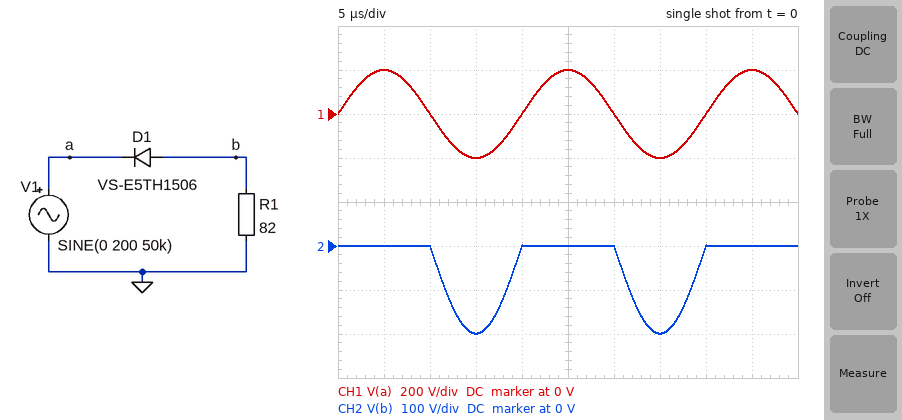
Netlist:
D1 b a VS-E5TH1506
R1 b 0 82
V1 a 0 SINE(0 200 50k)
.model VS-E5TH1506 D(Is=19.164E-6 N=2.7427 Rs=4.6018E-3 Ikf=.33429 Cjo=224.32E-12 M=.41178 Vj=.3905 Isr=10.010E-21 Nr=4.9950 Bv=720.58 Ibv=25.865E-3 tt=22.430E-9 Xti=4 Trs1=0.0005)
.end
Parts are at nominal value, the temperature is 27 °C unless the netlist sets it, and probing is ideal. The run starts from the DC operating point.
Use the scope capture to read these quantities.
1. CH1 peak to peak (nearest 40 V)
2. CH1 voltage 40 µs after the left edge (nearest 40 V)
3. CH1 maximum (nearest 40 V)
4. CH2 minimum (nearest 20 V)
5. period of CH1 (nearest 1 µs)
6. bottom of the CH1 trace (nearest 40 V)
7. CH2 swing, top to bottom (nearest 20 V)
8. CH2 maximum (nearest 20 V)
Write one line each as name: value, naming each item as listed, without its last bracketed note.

CH1 peak to peak: 400 V
CH1 voltage 40 µs after the left edge: 0 V
CH1 maximum: 200 V
CH2 minimum: -200 V
period of CH1: 20 µs
bottom of the CH1 trace: -200 V
CH2 swing, top to bottom: 200 V
CH2 maximum: 0 V
